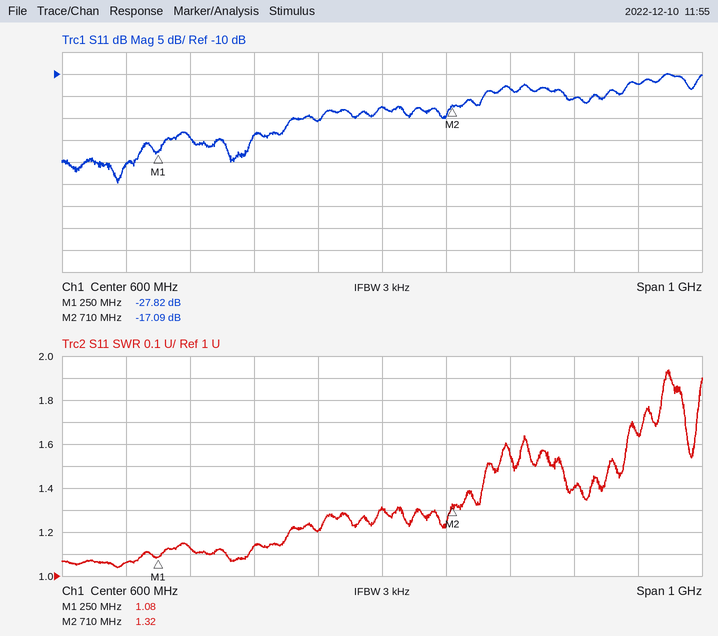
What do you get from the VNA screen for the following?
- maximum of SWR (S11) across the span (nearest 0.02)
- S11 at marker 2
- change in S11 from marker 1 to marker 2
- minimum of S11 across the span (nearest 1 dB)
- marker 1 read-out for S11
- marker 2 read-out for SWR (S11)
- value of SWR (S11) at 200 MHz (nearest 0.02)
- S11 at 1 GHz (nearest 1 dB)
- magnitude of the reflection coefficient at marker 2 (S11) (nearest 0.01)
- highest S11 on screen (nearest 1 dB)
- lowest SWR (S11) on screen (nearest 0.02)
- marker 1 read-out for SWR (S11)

1.94
-17.09 dB
10.73 dB
-35 dB
-27.82 dB
1.32
1.06
-12 dB
0.14
-10 dB
1.04
1.08
